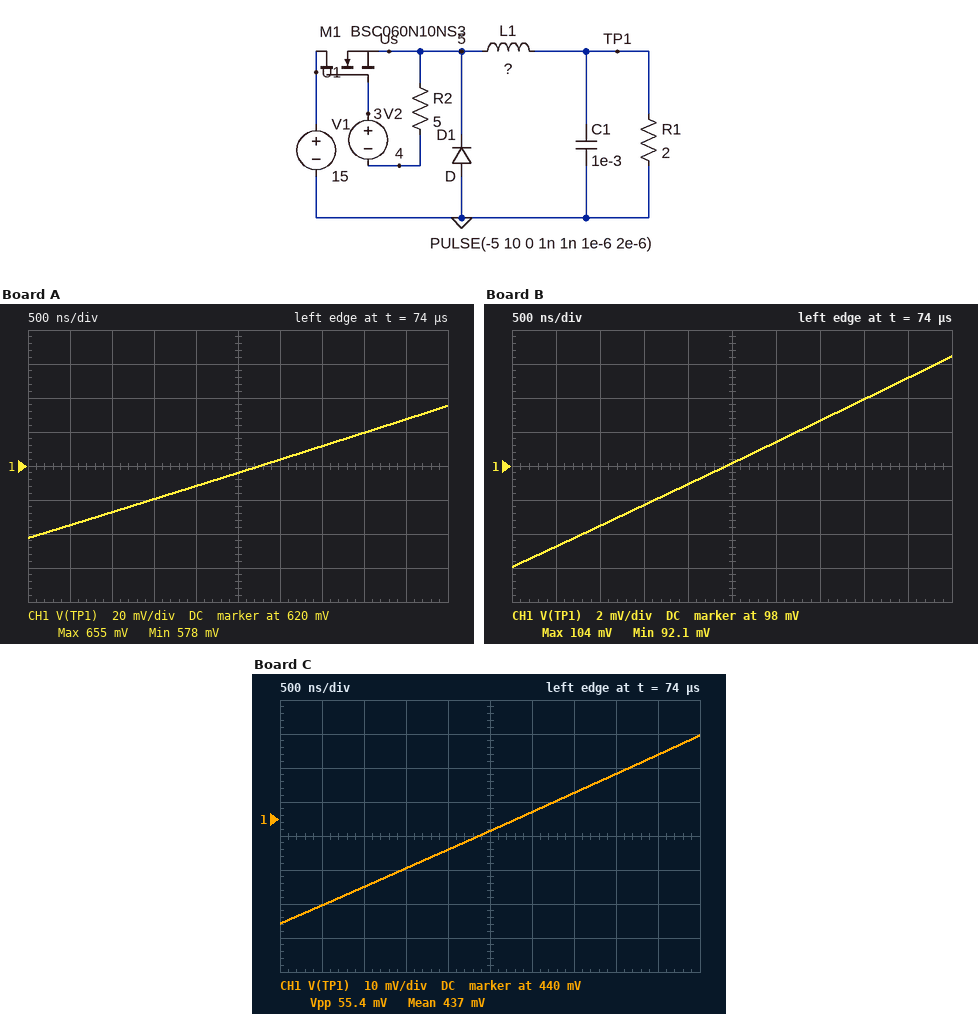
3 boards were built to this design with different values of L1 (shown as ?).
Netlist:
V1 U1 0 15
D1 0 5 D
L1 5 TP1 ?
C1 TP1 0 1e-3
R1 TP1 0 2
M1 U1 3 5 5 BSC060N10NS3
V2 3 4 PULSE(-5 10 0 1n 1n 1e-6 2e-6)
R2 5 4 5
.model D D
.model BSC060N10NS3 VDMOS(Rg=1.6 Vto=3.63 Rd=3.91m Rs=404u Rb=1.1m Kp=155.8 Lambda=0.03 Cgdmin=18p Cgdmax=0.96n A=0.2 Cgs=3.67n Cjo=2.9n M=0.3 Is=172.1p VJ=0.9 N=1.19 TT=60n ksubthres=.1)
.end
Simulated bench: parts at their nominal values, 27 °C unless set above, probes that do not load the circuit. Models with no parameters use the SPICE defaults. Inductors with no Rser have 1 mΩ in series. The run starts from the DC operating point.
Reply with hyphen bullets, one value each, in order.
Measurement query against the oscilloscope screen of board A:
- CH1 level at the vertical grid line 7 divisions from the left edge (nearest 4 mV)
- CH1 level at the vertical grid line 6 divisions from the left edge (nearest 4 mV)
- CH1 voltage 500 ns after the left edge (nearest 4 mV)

- 632 mV
- 624 mV
- 584 mV
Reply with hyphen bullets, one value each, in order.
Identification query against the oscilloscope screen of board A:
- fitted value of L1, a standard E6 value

- 33 µH
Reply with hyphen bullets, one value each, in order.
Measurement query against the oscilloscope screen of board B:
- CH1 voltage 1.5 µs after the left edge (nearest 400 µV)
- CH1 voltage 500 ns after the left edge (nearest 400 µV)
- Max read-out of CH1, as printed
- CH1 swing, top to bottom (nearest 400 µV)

- 95.6 mV
- 93.2 mV
- 104 mV
- 12.4 mV
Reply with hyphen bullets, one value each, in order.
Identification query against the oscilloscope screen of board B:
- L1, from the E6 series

- 220 µH
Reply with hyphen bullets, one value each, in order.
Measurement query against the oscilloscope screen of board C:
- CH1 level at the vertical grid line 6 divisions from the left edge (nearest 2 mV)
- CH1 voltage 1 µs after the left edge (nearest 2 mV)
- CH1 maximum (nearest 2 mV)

- 442 mV
- 420 mV
- 464 mV
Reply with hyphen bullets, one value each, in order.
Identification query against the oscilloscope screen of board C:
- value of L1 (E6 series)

- 47 µH
